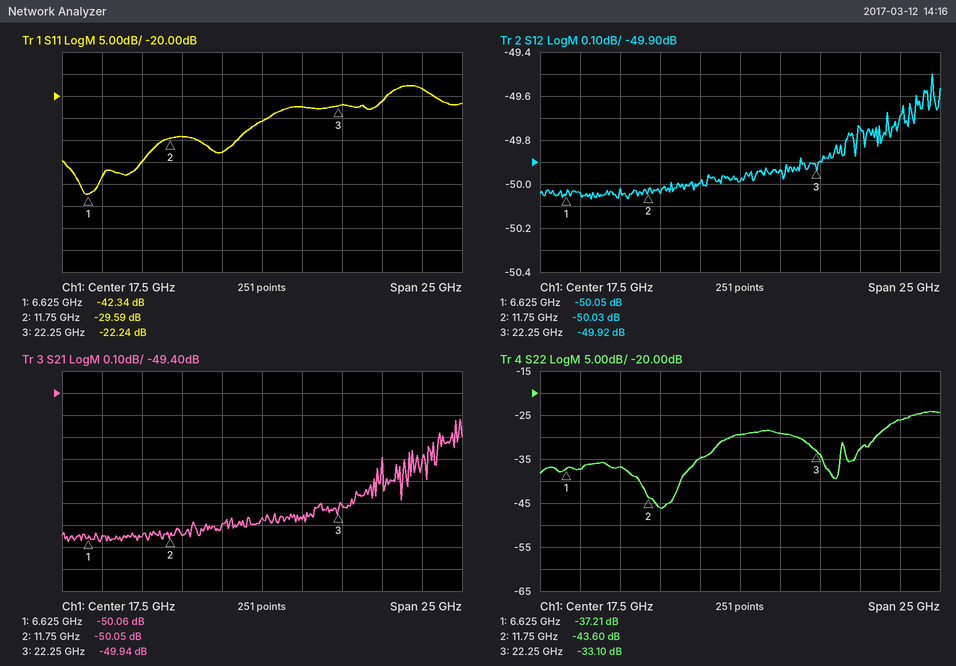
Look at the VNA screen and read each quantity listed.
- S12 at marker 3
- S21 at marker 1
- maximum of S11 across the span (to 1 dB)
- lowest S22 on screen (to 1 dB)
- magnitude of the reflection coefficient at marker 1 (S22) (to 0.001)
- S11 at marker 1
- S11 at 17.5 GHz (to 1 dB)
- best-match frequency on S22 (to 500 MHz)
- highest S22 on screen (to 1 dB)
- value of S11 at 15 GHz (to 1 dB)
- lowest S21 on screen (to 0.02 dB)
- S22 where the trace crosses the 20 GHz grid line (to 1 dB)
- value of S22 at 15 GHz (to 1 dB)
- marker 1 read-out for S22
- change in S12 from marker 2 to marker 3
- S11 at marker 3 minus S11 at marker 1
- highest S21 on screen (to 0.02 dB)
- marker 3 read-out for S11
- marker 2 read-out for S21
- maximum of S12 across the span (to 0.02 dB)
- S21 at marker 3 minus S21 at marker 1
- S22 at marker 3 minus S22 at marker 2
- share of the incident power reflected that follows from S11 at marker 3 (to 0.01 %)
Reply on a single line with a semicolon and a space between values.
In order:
-49.92 dB; -50.06 dB; -18 dB; -46 dB; 0.014; -42.34 dB; -26 dB; 12.5 GHz; -24 dB; -33 dB; -50.08 dB; -29 dB; -35 dB; -37.21 dB; 0.11 dB; 20.10 dB; -49.52 dB; -22.24 dB; -50.05 dB; -49.50 dB; 0.12 dB; 10.50 dB; 0.60 %
